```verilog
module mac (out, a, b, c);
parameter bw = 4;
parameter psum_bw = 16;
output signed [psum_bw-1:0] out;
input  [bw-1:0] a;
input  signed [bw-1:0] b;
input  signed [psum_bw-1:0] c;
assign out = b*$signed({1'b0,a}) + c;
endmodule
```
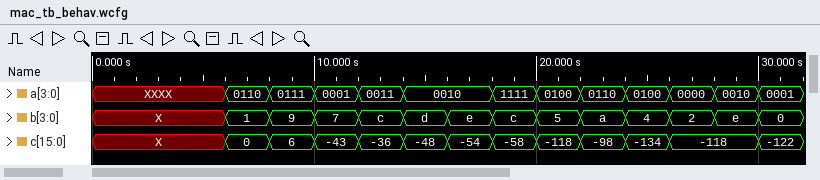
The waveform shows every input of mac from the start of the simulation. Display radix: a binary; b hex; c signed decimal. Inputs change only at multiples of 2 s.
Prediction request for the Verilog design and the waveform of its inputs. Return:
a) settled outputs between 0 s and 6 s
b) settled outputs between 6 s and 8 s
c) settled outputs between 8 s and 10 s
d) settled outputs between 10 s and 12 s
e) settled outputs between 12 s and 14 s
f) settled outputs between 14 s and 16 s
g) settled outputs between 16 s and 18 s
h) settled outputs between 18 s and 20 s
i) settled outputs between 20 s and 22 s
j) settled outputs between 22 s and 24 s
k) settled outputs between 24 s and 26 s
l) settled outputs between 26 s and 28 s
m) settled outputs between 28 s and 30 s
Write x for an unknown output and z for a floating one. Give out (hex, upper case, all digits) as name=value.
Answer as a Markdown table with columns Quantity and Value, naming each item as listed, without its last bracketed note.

| Quantity | Value |
|---|---|
| settled outputs between 0 s and 6 s | out=x |
| settled outputs between 6 s and 8 s | out=0006 |
| settled outputs between 8 s and 10 s | out=FFD5 |
| settled outputs between 10 s and 12 s | out=FFDC |
| settled outputs between 12 s and 14 s | out=FFD0 |
| settled outputs between 14 s and 16 s | out=FFCA |
| settled outputs between 16 s and 18 s | out=FFC6 |
| settled outputs between 18 s and 20 s | out=FF8A |
| settled outputs between 20 s and 22 s | out=FF9E |
| settled outputs between 22 s and 24 s | out=FF7A |
| settled outputs between 24 s and 26 s | out=FF8A |
| settled outputs between 26 s and 28 s | out=FF8A |
| settled outputs between 28 s and 30 s | out=FF86 |
